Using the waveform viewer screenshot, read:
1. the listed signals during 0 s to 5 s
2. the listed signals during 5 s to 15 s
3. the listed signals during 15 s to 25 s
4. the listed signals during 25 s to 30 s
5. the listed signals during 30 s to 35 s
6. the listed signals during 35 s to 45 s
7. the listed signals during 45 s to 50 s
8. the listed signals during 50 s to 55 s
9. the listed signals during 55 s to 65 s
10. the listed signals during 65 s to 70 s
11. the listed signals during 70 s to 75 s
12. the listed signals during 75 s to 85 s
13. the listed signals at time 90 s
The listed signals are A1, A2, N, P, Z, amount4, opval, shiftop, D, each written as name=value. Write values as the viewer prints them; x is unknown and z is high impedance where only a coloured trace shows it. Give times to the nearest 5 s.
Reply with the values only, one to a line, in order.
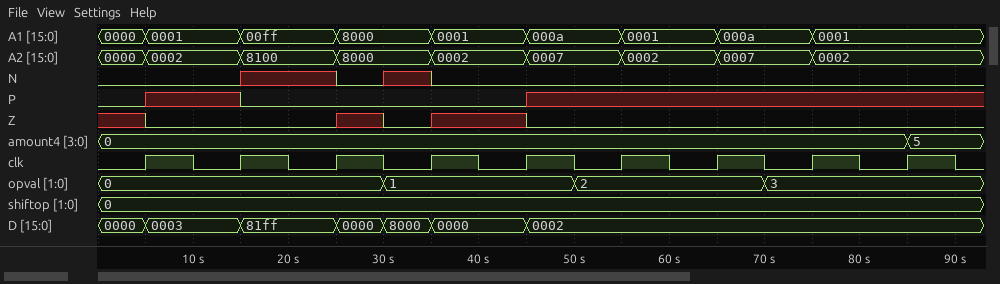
A1=0000, A2=0000, N=0, P=0, Z=x, amount4=0, opval=0, shiftop=0, D=0000
A1=0001, A2=0002, N=0, P=x, Z=0, amount4=0, opval=0, shiftop=0, D=0003
A1=00ff, A2=8100, N=x, P=0, Z=0, amount4=0, opval=0, shiftop=0, D=81ff
A1=8000, A2=8000, N=0, P=0, Z=x, amount4=0, opval=0, shiftop=0, D=0000
A1=8000, A2=8000, N=x, P=0, Z=0, amount4=0, opval=1, shiftop=0, D=8000
A1=0001, A2=0002, N=0, P=0, Z=x, amount4=0, opval=1, shiftop=0, D=0000
A1=000a, A2=0007, N=0, P=x, Z=0, amount4=0, opval=1, shiftop=0, D=0002
A1=000a, A2=0007, N=0, P=x, Z=0, amount4=0, opval=2, shiftop=0, D=0002
A1=0001, A2=0002, N=0, P=x, Z=0, amount4=0, opval=2, shiftop=0, D=0002
A1=000a, A2=0007, N=0, P=x, Z=0, amount4=0, opval=2, shiftop=0, D=0002
A1=000a, A2=0007, N=0, P=x, Z=0, amount4=0, opval=3, shiftop=0, D=0002
A1=0001, A2=0002, N=0, P=x, Z=0, amount4=0, opval=3, shiftop=0, D=0002
A1=0001, A2=0002, N=0, P=x, Z=0, amount4=5, opval=3, shiftop=0, D=0002
